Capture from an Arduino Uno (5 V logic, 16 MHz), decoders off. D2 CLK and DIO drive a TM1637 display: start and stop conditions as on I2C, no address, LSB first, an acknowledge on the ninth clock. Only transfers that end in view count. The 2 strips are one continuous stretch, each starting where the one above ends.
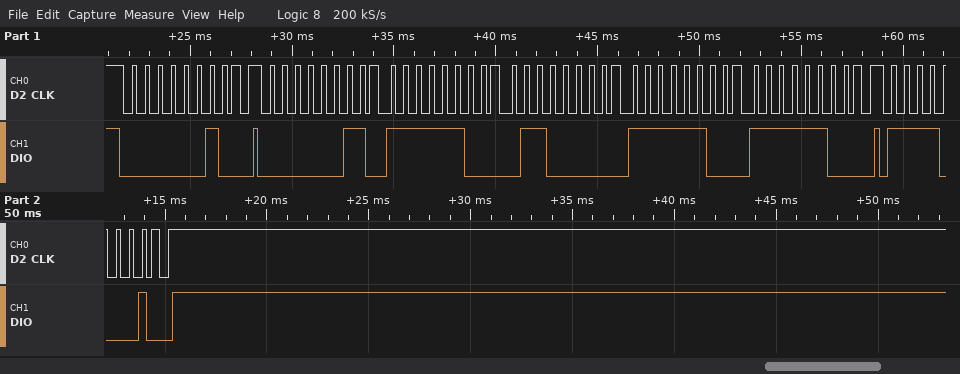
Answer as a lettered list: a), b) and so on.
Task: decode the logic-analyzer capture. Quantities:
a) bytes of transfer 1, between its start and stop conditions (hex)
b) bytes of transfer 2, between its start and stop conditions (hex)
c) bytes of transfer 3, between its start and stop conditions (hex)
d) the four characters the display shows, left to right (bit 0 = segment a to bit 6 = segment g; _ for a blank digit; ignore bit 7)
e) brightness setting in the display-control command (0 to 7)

a) 40
b) C0 3F 06 3F 3F
c) 8F
d) 0100
e) 7
